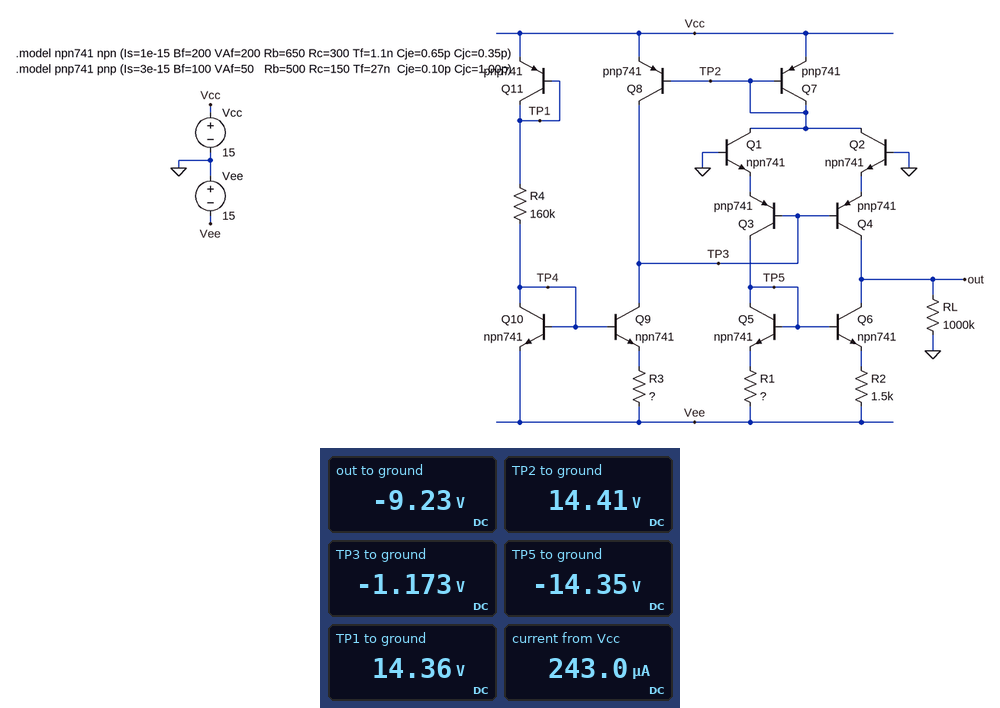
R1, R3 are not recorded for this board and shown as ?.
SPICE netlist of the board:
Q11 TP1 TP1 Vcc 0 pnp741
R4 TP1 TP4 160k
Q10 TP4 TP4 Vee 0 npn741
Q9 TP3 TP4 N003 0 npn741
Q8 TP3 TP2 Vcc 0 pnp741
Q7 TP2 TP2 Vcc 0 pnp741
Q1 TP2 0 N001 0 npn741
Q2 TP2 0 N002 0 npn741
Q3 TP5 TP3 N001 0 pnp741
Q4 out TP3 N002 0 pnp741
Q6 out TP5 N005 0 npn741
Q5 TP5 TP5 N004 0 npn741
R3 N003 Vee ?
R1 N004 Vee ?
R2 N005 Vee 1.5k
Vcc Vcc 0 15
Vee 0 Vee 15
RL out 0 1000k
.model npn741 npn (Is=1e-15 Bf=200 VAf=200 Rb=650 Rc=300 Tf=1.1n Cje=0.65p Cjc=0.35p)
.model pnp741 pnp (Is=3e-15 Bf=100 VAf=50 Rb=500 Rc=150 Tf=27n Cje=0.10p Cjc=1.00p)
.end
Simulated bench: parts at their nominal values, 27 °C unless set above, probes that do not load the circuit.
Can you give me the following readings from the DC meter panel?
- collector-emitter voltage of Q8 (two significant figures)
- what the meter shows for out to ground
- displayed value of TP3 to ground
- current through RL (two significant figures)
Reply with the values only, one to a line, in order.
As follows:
-16 V
-9.23 V
-1.173 V
9.2 µA
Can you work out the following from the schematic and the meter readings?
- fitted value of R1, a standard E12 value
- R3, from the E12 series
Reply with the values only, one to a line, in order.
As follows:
3.3 kΩ
1.2 kΩ
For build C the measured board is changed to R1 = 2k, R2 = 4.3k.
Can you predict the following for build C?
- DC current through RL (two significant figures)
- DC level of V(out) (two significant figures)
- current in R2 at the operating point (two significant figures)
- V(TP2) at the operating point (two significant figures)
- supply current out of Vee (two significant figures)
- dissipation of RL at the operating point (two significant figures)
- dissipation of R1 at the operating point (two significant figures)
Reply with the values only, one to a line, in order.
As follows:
640 nA
-640 mV
9.6 µA
14 V
240 µA
410 nW
420 nW
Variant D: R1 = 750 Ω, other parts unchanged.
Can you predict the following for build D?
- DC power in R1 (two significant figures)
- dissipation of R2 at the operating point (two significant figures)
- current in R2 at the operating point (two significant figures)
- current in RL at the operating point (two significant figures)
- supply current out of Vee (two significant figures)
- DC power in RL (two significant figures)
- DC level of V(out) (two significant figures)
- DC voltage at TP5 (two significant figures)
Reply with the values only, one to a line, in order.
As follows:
160 nW
210 nW
12 µA
670 nA
240 µA
440 nW
-670 mV
-14 V
